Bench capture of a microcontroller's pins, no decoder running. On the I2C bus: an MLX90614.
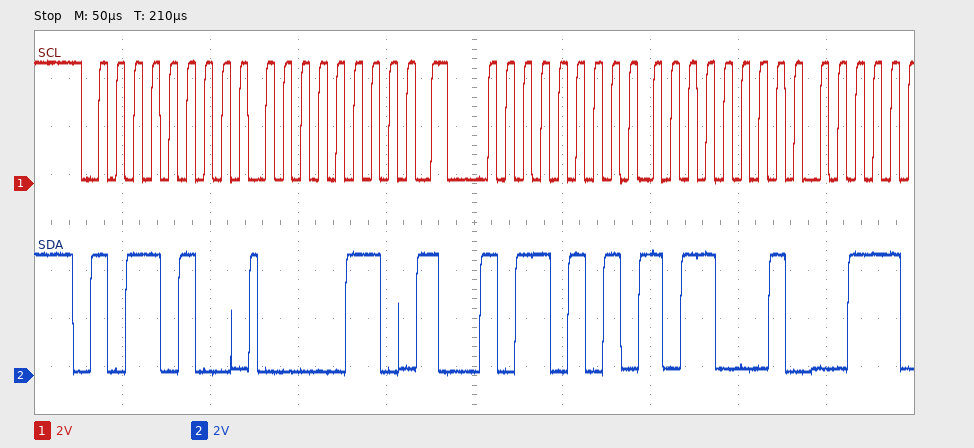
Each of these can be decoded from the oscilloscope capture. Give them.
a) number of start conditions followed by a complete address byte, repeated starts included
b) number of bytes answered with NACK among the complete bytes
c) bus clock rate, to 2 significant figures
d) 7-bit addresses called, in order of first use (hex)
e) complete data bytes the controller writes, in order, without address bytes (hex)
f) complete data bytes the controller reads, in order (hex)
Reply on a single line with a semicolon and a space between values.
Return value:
2; 0; 100 kHz; 0x5A; 06; B1
